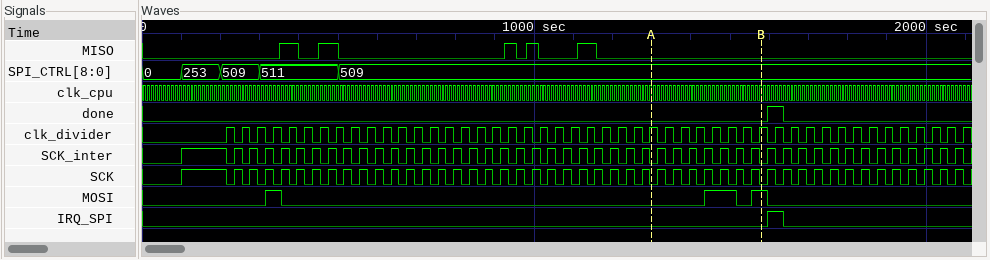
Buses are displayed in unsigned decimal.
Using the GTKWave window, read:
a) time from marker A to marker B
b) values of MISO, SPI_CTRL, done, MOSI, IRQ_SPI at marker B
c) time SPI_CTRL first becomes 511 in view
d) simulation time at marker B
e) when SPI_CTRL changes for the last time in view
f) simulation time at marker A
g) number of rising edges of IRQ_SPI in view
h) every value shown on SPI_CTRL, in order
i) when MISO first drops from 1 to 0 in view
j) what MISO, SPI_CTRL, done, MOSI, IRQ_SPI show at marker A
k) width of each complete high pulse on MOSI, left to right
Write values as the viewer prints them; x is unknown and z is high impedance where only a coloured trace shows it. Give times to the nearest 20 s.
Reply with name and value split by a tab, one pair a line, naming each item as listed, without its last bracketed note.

time from marker A to marker B	280 s
values of MISO, SPI_CTRL, done, MOSI, IRQ_SPI at marker B	MISO=0, SPI_CTRL=509, done=0, MOSI=1, IRQ_SPI=0
time SPI_CTRL first becomes 511 in view	300 s
simulation time at marker B	1580 s
when SPI_CTRL changes for the last time in view	500 s
simulation time at marker A	1300 s
number of rising edges of IRQ_SPI in view	1
every value shown on SPI_CTRL, in order	0, 253, 509, 511, 509
when MISO first drops from 1 to 0 in view	400 s
what MISO, SPI_CTRL, done, MOSI, IRQ_SPI show at marker A	MISO=0, SPI_CTRL=509, done=0, MOSI=0, IRQ_SPI=0
width of each complete high pulse on MOSI, left to right	40 s, 80 s, 40 s
